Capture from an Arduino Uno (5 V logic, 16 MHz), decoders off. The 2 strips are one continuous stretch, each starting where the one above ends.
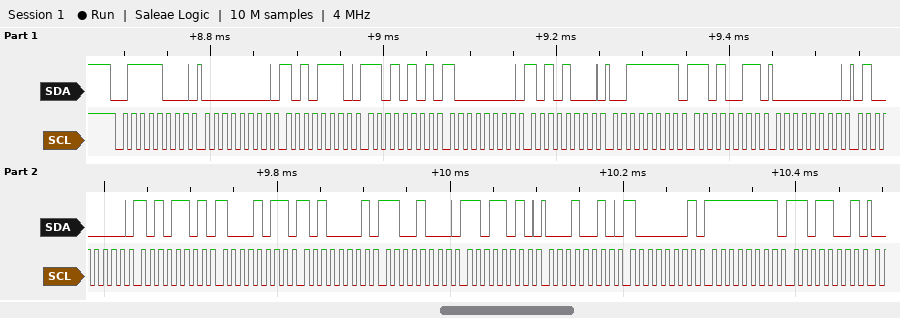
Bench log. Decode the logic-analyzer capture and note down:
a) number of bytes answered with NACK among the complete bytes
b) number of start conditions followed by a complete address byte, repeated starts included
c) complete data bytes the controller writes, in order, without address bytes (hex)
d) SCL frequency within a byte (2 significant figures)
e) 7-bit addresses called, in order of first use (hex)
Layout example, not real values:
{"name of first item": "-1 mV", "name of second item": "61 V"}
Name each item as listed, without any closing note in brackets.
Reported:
{"number of bytes answered with NACK among the complete bytes": "0", "number of start conditions followed by a complete address byte, repeated starts included": "1", "complete data bytes the controller writes, in order, without address bytes": "00 AE D5 80 A8 3F D3 00 40 AD 8B A1 C8 DA 12 81 FF D9", "SCL frequency within a byte": "100 kHz", "7-bit addresses called, in order of first use": "0x3C"}
